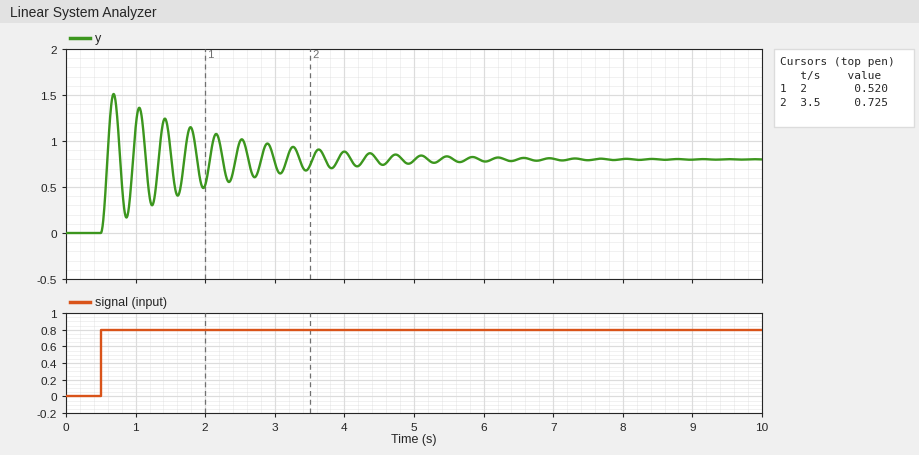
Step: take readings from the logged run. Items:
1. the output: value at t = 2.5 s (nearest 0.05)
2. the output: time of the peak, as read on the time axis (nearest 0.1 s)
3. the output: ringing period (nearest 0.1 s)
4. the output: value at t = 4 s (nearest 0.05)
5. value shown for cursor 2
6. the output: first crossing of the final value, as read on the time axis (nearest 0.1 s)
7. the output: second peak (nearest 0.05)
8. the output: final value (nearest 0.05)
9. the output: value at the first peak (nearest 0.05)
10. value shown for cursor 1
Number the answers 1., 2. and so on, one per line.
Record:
1. 1.00
2. 0.7 s
3. 0.4 s
4. 0.90
5. 0.725
6. 0.6 s
7. 1.35
8. 0.80
9. 1.50
10. 0.520
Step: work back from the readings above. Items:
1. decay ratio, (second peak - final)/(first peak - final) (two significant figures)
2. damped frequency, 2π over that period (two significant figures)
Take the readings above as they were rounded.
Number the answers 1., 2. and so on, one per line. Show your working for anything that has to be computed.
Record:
1. (1.35 - 0.8) / (1.5 - 0.8) = 0.79
2. 2π / 0.4 = 16 rad/s
